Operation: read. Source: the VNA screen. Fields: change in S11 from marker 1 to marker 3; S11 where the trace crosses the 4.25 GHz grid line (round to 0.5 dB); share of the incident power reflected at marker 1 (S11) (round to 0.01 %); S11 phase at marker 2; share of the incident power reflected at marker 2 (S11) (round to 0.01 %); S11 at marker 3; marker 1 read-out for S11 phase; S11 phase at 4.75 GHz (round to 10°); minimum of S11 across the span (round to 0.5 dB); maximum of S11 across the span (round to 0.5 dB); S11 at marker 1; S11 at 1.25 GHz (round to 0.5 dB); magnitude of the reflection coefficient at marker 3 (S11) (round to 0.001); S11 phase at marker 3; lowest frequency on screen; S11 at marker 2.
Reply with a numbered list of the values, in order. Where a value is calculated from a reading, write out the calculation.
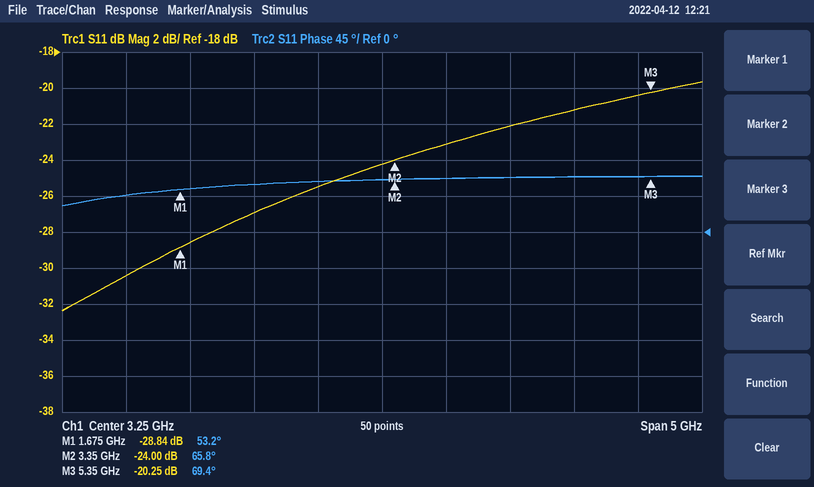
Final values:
1. -20.25 − (-28.84) = 8.59 dB
2. -22.0 dB
3. 10^(-28.84/10) ≈ 0.13 %
4. 65.8°
5. 10^(-24/10) ≈ 0.40 %
6. -20.25 dB
7. 53.2°
8. 70°
9. -32.5 dB
10. -19.5 dB
11. -28.84 dB
12. -30.5 dB
13. 10^(-20.25/20) ≈ 0.097
14. 69.4°
15. 750 MHz
16. -24.00 dB
